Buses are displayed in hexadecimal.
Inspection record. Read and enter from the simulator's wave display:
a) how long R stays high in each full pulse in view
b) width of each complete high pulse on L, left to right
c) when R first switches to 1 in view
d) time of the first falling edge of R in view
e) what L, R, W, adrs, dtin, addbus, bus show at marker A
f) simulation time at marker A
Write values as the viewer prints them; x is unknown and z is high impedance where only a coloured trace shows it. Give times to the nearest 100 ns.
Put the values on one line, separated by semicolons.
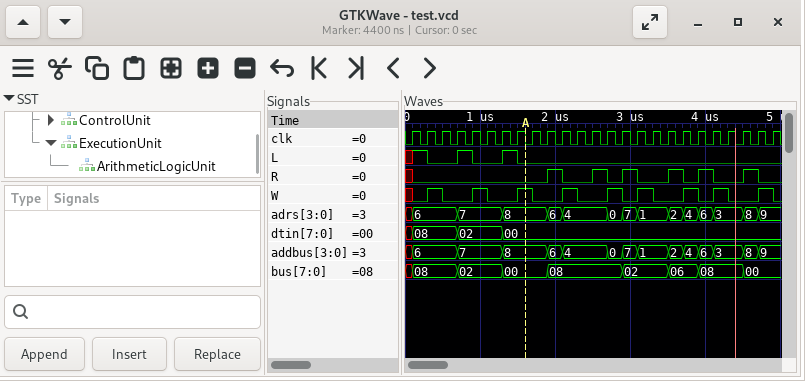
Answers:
200 ns, 200 ns, 200 ns, 200 ns, 200 ns, 200 ns; 200 ns, 200 ns; 1900 ns; 2100 ns; L=0, R=0, W=1, adrs=8, dtin=00, addbus=8, bus=00; 1600 ns
